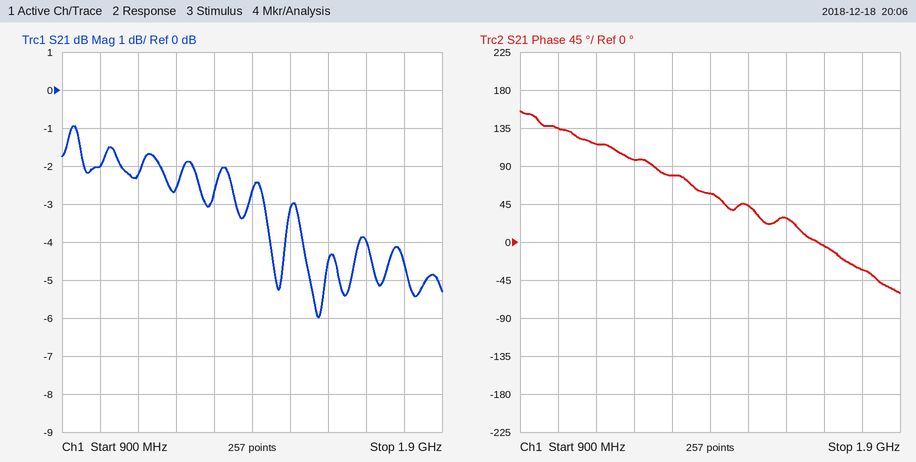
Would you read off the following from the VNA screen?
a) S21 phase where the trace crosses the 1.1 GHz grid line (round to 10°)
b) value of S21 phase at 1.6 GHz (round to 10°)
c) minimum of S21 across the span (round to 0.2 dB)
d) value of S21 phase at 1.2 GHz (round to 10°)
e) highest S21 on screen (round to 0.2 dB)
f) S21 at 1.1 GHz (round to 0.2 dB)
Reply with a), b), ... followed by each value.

a) 120°
b) 30°
c) -6.0 dB
d) 100°
e) -1.0 dB
f) -2.2 dB
